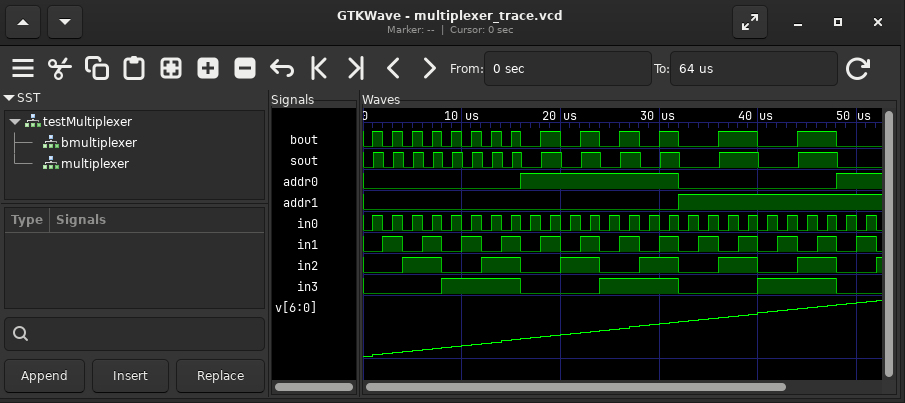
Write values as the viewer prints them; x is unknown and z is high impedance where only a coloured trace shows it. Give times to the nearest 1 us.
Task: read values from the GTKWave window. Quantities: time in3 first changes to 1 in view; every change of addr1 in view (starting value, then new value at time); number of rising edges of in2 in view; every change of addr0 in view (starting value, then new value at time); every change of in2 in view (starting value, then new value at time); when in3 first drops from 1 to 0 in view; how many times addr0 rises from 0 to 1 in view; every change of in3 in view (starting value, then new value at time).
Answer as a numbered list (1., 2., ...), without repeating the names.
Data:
1. 8 us
2. 0, 1 at 32 us
3. 7
4. 0, 1 at 16 us, 0 at 32 us, 1 at 48 us
5. 0, 1 at 4 us, 0 at 8 us, 1 at 12 us, 0 at 16 us, 1 at 20 us, 0 at 24 us, 1 at 28 us, 0 at 32 us, 1 at 36 us, 0 at 40 us, 1 at 44 us, 0 at 48 us, 1 at 52 us
6. 16 us
7. 2
8. 0, 1 at 8 us, 0 at 16 us, 1 at 24 us, 0 at 32 us, 1 at 40 us, 0 at 48 us
